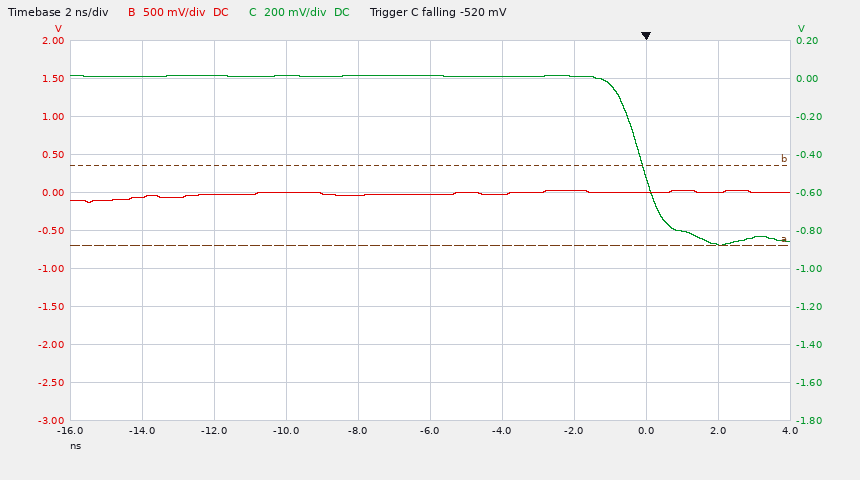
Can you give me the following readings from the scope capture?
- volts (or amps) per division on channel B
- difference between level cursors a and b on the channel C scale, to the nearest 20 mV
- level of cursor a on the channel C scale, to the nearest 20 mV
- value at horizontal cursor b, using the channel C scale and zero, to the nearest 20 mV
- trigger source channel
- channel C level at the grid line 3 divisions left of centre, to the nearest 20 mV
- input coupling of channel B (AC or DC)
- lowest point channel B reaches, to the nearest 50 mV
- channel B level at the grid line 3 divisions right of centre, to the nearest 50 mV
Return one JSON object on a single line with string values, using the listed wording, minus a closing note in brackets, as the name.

{"volts (or amps) per division on channel B": "500 mV", "difference between level cursors a and b on the channel C scale, to the nearest 20 mV": "420 mV", "level of cursor a on the channel C scale, to the nearest 20 mV": "-880 mV", "value at horizontal cursor b, using the channel C scale and zero, to the nearest 20 mV": "-460 mV", "trigger source channel": "channel C", "channel C level at the grid line 3 divisions left of centre, to the nearest 20 mV": "20 mV", "input coupling of channel B": "DC", "lowest point channel B reaches, to the nearest 50 mV": "-150 mV", "channel B level at the grid line 3 divisions right of centre, to the nearest 50 mV": "0 mV"}
